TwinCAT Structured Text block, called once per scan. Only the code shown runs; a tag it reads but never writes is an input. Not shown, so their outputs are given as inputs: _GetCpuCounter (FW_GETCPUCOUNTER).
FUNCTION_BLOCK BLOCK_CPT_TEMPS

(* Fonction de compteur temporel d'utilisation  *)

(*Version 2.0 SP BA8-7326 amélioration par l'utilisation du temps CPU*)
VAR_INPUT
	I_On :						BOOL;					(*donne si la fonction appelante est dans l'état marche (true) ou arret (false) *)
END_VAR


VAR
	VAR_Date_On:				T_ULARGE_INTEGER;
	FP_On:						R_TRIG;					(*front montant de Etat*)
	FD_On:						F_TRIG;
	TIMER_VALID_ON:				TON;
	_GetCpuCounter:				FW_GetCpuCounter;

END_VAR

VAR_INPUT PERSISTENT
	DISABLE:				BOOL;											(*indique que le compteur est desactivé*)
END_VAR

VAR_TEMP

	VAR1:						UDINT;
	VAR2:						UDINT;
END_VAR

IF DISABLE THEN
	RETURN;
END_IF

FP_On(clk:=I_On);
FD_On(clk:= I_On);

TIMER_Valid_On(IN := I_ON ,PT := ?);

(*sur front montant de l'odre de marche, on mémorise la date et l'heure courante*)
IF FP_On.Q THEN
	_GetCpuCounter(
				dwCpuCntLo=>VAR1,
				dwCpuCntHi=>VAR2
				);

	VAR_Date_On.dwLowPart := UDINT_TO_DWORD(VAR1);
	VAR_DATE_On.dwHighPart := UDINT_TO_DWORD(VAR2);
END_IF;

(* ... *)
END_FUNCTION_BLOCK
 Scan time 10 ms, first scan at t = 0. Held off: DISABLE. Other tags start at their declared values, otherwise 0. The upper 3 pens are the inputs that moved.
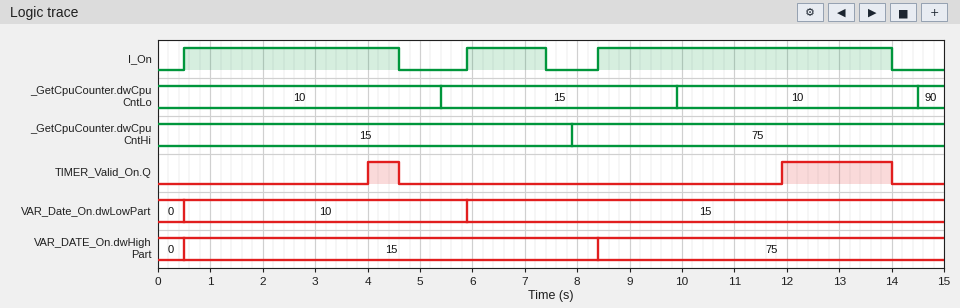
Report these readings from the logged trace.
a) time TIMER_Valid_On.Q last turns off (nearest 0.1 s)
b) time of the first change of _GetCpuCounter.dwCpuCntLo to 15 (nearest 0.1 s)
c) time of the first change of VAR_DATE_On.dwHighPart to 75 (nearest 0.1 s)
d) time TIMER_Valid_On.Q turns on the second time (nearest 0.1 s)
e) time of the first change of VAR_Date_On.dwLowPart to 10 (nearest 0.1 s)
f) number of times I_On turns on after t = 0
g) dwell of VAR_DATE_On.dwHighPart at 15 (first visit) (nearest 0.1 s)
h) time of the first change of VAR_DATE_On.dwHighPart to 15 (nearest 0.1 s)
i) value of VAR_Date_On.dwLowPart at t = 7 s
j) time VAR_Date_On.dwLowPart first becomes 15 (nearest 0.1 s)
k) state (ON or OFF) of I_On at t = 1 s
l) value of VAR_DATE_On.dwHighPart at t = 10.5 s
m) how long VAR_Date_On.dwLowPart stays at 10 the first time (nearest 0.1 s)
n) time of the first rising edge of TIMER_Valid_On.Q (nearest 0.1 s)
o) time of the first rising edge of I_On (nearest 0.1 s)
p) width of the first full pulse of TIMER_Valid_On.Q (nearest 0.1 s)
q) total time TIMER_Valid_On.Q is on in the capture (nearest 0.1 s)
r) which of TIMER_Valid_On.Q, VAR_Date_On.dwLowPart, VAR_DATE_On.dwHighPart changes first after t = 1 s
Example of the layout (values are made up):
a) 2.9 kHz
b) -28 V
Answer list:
a) 14.0 s
b) 5.4 s
c) 8.4 s
d) 11.9 s
e) 0.5 s
f) 3
g) 7.9 s
h) 0.5 s
i) 15
j) 5.9 s
k) ON
l) 75
m) 5.4 s
n) 4.0 s
o) 0.5 s
p) 0.6 s
q) 2.7 s
r) TIMER_Valid_On.Q
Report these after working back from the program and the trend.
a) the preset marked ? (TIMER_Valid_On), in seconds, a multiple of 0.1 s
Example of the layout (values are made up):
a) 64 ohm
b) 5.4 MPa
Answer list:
a) 3.5 s
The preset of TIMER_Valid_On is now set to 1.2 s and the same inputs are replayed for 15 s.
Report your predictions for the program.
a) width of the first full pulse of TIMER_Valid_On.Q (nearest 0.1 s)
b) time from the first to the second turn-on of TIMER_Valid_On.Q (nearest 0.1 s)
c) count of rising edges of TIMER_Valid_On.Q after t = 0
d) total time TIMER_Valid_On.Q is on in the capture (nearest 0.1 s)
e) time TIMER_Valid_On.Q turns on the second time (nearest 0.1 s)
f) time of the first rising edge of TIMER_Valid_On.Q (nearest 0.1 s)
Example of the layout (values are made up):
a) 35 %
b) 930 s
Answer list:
a) 2.9 s
b) 5.4 s
c) 3
d) 7.6 s
e) 7.1 s
f) 1.7 s
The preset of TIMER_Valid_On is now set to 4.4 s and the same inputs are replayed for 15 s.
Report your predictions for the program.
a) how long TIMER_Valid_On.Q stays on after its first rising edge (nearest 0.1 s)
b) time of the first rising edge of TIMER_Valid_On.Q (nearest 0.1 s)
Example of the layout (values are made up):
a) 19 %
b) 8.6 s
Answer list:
a) 1.2 s
b) 12.8 s
